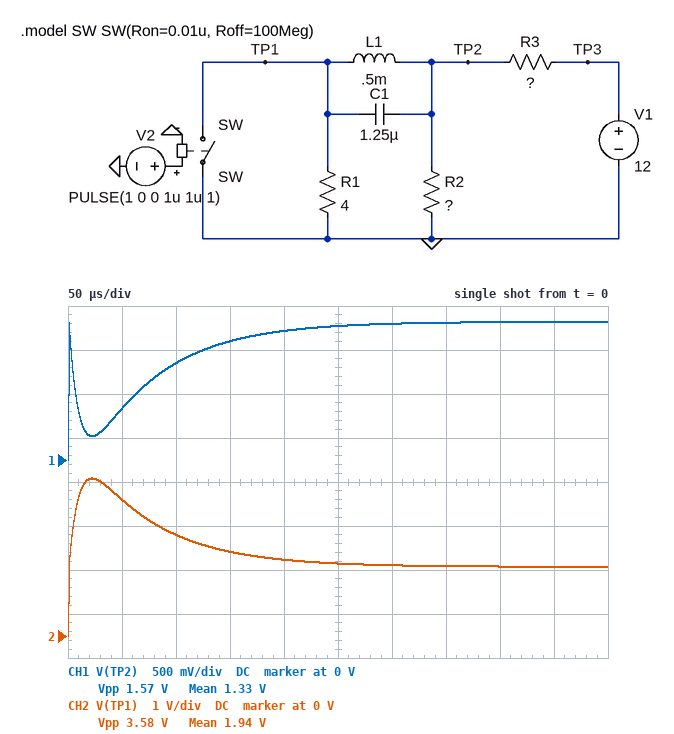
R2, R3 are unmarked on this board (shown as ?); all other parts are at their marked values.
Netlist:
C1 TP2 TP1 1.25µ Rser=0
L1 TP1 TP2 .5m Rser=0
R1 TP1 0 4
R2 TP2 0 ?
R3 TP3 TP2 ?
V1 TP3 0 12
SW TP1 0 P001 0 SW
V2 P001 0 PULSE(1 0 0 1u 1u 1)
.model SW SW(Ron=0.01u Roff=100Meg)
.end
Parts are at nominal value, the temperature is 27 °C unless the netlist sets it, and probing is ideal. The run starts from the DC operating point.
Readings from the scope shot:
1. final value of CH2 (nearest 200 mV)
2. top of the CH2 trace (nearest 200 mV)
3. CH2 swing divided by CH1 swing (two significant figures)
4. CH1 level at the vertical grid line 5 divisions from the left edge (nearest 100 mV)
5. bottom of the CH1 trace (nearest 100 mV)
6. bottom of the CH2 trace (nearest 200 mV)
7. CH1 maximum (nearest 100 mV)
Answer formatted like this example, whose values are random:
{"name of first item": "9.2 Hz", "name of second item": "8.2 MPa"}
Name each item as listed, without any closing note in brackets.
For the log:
{"final value of CH2": "1.6 V", "top of the CH2 trace": "3.6 V", "CH2 swing divided by CH1 swing": "2.3", "CH1 level at the vertical grid line 5 divisions from the left edge": "1.5 V", "bottom of the CH1 trace": "0 V", "bottom of the CH2 trace": "0 V", "CH1 maximum": "1.6 V"}
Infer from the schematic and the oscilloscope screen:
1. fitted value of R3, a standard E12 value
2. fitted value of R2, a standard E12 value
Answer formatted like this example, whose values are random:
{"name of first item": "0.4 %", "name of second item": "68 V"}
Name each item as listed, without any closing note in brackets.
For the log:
{"fitted value of R3, a standard E12 value": "12 Ω", "fitted value of R2, a standard E12 value": "3.3 Ω"}
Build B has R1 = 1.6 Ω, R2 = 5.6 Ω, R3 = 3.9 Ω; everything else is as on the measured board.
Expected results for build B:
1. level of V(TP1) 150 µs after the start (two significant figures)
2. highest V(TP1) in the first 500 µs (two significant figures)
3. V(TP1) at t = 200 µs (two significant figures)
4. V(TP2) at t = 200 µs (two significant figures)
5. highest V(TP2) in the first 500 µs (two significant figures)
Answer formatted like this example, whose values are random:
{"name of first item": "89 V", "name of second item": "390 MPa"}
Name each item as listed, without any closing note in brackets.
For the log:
{"level of V(TP1) 150 µs after the start": "3.6 V", "highest V(TP1) in the first 500 µs": "4.7 V", "V(TP1) at t = 200 µs": "3.3 V", "V(TP2) at t = 200 µs": "2.3 V", "highest V(TP2) in the first 500 µs": "2.9 V"}
